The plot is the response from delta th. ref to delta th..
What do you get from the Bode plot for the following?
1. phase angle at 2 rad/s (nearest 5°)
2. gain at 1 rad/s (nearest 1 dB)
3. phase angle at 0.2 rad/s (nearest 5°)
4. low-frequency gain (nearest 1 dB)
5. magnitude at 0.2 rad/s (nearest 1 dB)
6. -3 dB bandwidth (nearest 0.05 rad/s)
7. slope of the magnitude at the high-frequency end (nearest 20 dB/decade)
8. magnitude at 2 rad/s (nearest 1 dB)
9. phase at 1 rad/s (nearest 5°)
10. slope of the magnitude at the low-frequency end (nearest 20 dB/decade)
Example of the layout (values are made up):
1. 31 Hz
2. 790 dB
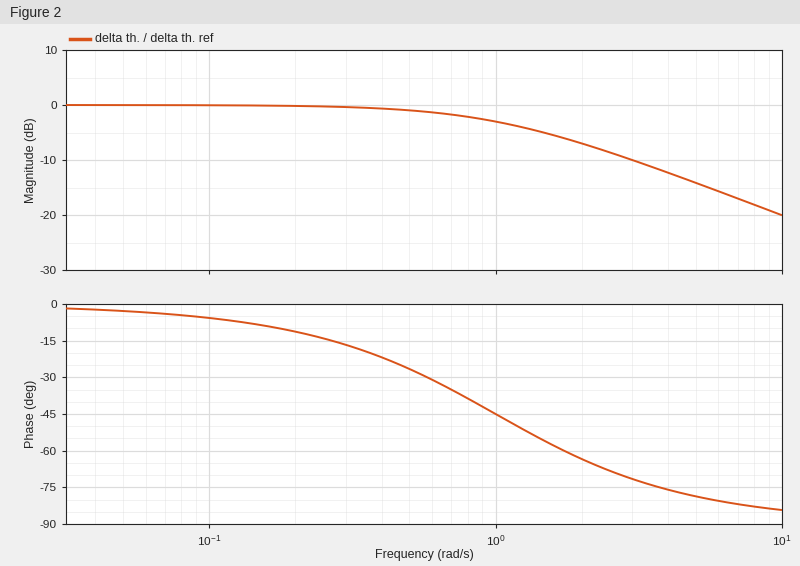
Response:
1. -65°
2. -3 dB
3. -10°
4. 0 dB
5. 0 dB
6. 1.00 rad/s
7. -20 dB/decade
8. -7 dB
9. -45°
10. 0 dB/decade
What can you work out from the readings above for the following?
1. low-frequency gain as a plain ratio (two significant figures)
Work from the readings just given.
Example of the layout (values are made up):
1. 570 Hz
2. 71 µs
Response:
1. 1.0
